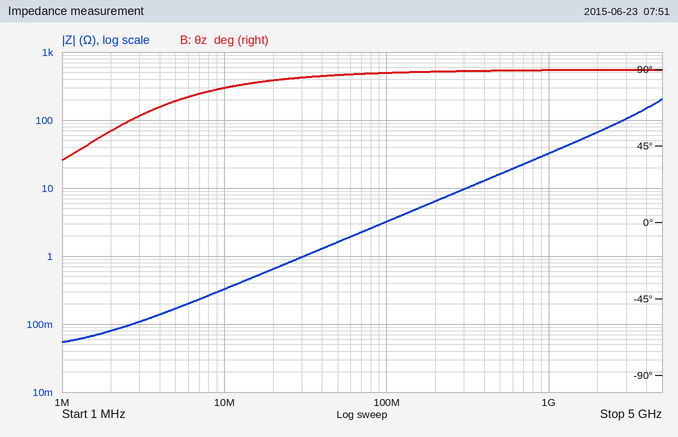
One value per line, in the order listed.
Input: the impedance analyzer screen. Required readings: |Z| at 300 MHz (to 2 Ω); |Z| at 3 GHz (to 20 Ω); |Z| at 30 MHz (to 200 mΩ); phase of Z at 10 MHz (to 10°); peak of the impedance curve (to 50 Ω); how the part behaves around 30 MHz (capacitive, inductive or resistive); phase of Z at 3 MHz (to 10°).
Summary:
10 Ω
100 Ω
1.0 Ω
80°
200 Ω
inductive
60°
